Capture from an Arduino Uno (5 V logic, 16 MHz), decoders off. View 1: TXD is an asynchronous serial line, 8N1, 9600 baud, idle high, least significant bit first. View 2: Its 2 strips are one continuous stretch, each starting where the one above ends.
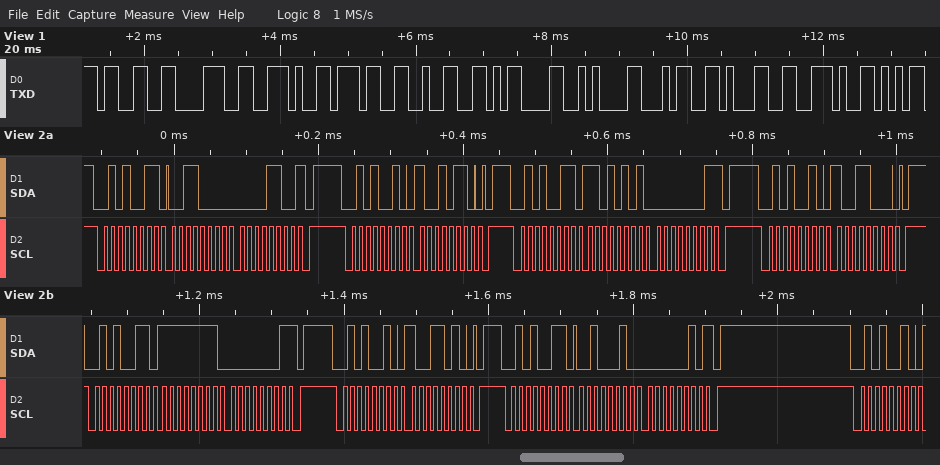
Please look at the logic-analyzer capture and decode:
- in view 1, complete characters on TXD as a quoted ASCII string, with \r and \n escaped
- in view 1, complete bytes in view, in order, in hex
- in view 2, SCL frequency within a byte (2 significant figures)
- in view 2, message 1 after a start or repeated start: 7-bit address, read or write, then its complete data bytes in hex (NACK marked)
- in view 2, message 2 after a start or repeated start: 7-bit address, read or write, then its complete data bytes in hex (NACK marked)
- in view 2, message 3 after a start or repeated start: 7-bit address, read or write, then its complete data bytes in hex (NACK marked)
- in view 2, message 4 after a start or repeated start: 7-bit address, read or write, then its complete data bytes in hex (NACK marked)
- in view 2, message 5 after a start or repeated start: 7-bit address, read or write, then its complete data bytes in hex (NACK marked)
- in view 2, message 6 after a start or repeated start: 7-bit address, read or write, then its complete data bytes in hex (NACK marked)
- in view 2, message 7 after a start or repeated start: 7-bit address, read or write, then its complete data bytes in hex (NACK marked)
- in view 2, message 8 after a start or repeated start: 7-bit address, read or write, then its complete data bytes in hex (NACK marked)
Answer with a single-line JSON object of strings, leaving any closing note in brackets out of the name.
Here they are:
{"in view 1, complete characters on TXD as a quoted ASCII string, with \\r and \\n escaped": "\"38.72\\r\\n41.\"", "in view 1, complete bytes in view, in order, in hex": "33 38 2E 37 32 0D 0A 34 31 2E", "in view 2, SCL frequency within a byte": "100 kHz", "in view 2, message 1 after a start or repeated start: 7-bit address, read or write, then its complete data bytes in hex": "0x29 read: 30 0C NACK", "in view 2, message 2 after a start or repeated start: 7-bit address, read or write, then its complete data bytes in hex": "0x29 write: 96", "in view 2, message 3 after a start or repeated start: 7-bit address, read or write, then its complete data bytes in hex": "0x29 read: D5 01 NACK", "in view 2, message 4 after a start or repeated start: 7-bit address, read or write, then its complete data bytes in hex": "0x29 write: 98", "in view 2, message 5 after a start or repeated start: 7-bit address, read or write, then its complete data bytes in hex": "0x29 read: FF 01 NACK", "in view 2, message 6 after a start or repeated start: 7-bit address, read or write, then its complete data bytes in hex": "0x29 write: 9A", "in view 2, message 7 after a start or repeated start: 7-bit address, read or write, then its complete data bytes in hex": "0x29 read: 22 02 NACK", "in view 2, message 8 after a start or repeated start: 7-bit address, read or write, then its complete data bytes in hex": "0x29 write"}
